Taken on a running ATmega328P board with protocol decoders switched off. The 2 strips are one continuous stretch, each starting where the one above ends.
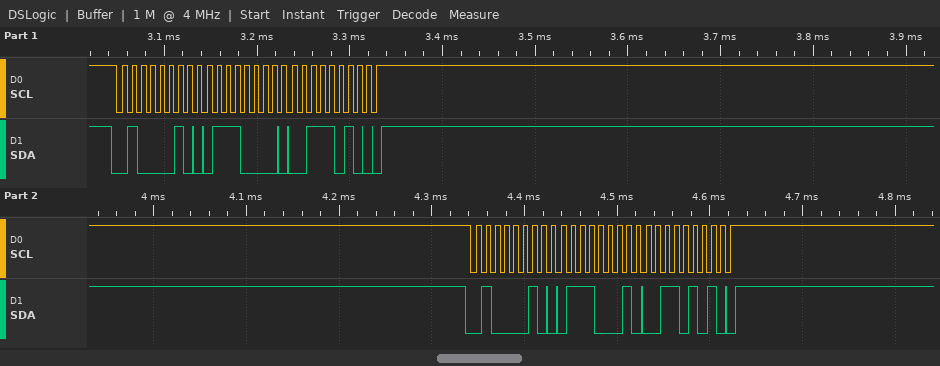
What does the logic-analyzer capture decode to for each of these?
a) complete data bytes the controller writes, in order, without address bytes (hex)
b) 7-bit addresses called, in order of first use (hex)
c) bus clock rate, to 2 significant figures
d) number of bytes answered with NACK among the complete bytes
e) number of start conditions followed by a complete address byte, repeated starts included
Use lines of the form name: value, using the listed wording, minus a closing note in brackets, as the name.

complete data bytes the controller writes, in order, without address bytes: 70 3A 71 35
7-bit addresses called, in order of first use: 0x21
bus clock rate, to 2 significant figures: 100 kHz
number of bytes answered with NACK among the complete bytes: 0
number of start conditions followed by a complete address byte, repeated starts included: 2
